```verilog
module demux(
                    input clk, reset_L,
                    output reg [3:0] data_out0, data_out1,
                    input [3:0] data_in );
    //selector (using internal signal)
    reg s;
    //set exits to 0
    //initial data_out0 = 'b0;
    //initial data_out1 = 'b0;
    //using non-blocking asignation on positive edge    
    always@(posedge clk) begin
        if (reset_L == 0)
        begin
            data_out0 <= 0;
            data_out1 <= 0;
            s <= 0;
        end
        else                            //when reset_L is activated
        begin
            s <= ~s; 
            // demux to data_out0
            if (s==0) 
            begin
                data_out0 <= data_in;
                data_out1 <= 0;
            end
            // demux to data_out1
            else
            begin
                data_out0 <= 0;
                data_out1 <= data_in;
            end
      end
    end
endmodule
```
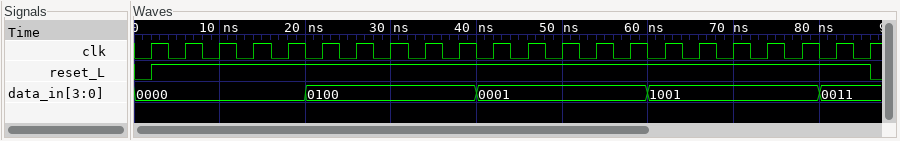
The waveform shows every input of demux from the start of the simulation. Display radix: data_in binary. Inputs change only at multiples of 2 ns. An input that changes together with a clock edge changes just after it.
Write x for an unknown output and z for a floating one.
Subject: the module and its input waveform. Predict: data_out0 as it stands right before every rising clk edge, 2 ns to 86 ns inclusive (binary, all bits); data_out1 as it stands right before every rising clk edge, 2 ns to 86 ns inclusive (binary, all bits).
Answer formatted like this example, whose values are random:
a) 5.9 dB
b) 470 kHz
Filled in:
a) x, 0000, 0000, 0000, 0000, 0000, 0100, 0000, 0100, 0000, 0100, 0000, 0001, 0000, 0001, 0000, 1001, 0000, 1001, 0000, 1001, 0000
b) x, 0000, 0000, 0000, 0000, 0000, 0000, 0100, 0000, 0100, 0000, 0001, 0000, 0001, 0000, 0001, 0000, 1001, 0000, 1001, 0000, 0011
